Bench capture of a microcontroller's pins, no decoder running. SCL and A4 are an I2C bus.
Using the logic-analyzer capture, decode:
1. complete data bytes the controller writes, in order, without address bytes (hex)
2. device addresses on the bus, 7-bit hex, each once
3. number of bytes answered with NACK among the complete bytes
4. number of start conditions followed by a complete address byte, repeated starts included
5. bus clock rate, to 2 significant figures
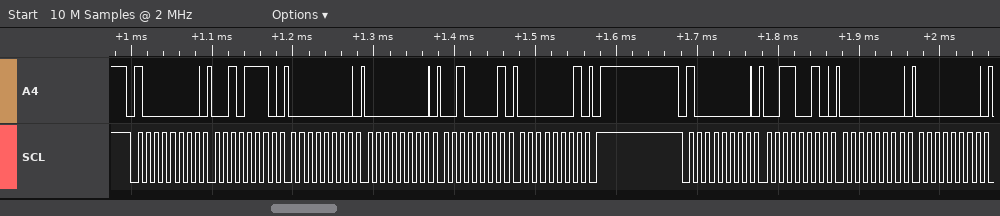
2E 00 00 21 01 32 00 00
0x40
0
2
100 kHz
